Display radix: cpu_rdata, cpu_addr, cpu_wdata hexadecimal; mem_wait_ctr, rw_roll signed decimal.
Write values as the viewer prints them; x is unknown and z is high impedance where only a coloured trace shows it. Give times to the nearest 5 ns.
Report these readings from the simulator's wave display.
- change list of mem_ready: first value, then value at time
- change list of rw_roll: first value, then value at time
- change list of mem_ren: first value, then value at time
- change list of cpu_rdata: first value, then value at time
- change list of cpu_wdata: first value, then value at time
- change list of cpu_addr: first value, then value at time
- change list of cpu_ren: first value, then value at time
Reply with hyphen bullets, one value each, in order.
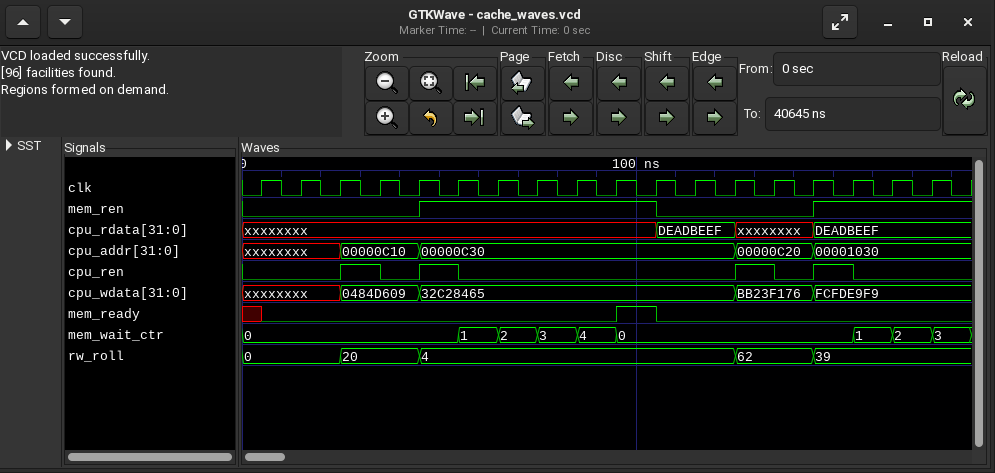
- x, 0 at 5 ns, 1 at 95 ns, 0 at 105 ns
- 0, 20 at 25 ns, 4 at 45 ns, 62 at 125 ns, 39 at 145 ns
- 0, 1 at 45 ns, 0 at 105 ns, 1 at 145 ns
- xxxxxxxx, DEADBEEF at 105 ns, xxxxxxxx at 125 ns, DEADBEEF at 145 ns
- xxxxxxxx, 0484D609 at 25 ns, 32C28465 at 45 ns, BB23F176 at 125 ns, FCFDE9F9 at 145 ns
- xxxxxxxx, 00000C10 at 25 ns, 00000C30 at 45 ns, 00000C20 at 125 ns, 00001030 at 145 ns
- 0, 1 at 25 ns, 0 at 35 ns, 1 at 45 ns, 0 at 55 ns, 1 at 125 ns, 0 at 135 ns, 1 at 145 ns, 0 at 155 ns
